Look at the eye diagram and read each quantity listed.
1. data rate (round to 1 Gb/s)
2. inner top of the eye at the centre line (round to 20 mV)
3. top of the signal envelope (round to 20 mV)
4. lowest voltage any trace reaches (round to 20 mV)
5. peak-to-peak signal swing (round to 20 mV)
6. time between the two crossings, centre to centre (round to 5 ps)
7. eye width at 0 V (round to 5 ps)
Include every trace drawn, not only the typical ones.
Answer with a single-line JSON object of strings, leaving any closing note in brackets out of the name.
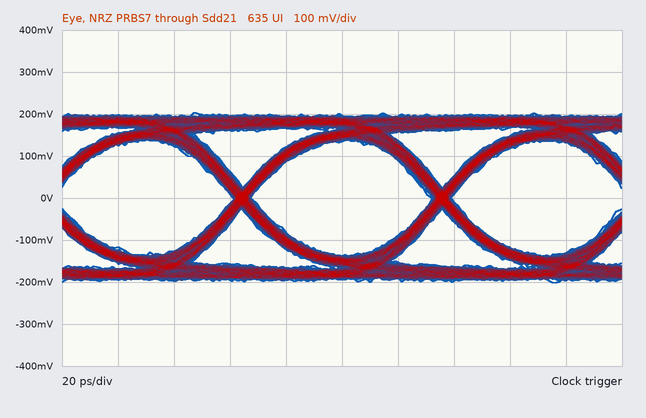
{"data rate": "14 Gb/s", "inner top of the eye at the centre line": "140 mV", "top of the signal envelope": "200 mV", "lowest voltage any trace reaches": "-200 mV", "peak-to-peak signal swing": "400 mV", "time between the two crossings, centre to centre": "70 ps", "eye width at 0 V": "65 ps"}
